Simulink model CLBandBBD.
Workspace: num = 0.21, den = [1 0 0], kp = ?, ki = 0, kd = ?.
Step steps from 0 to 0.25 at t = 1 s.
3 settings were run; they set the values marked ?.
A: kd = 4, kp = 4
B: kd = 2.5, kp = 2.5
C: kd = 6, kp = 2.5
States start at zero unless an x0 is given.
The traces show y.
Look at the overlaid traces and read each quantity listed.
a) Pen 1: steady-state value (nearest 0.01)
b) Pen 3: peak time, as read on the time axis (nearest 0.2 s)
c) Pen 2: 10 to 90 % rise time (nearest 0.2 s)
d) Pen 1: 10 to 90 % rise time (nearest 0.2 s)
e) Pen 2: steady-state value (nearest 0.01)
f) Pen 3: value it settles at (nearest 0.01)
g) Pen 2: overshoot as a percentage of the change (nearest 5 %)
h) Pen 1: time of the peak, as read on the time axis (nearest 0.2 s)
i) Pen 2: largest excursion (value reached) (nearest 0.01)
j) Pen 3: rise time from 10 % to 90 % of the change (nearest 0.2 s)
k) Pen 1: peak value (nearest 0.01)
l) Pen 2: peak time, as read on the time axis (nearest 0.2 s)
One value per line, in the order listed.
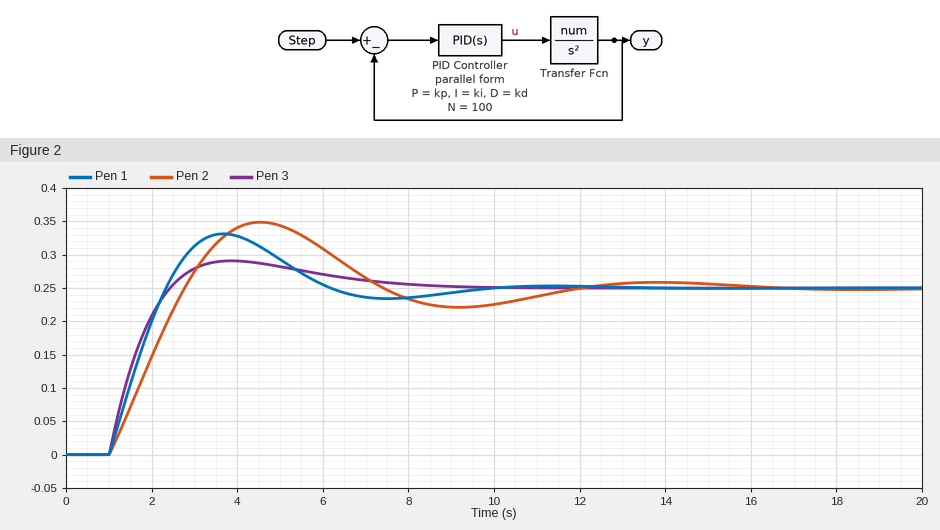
0.25
3.8 s
1.4 s
1.0 s
0.25
0.25
40 %
3.6 s
0.35
1.0 s
0.33
4.6 s
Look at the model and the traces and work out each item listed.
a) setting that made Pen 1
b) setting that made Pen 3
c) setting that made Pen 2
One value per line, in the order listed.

A
C
B
